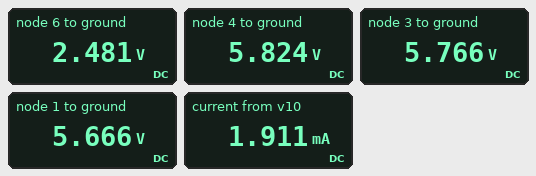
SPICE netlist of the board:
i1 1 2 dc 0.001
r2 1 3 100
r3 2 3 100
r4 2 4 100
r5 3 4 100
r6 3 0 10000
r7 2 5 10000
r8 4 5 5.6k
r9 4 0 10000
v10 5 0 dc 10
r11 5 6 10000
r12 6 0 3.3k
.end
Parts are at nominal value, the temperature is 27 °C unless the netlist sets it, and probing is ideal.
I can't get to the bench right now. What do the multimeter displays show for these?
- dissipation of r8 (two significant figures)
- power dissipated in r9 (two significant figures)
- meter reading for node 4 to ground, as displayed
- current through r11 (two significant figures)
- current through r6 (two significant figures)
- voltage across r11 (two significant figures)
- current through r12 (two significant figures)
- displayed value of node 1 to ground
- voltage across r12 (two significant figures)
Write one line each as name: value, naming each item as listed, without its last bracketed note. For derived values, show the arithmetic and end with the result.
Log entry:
dissipation of r8: (10 V - 5.824 V)^2 / 5.6 kΩ = 3.1 mW
power dissipated in r9: (5.824 V)^2 / 10 kΩ = 3.4 mW
meter reading for node 4 to ground, as displayed: 5.824 V
current through r11: (10 V - 2.481 V) / 10 kΩ = 750 µA
current through r6: (5.766 V) / 10 kΩ = 580 µA
voltage across r11: 10 V - 2.481 V = 7.5 V
current through r12: (2.481 V) / 3.3 kΩ = 750 µA
displayed value of node 1 to ground: 5.666 V
voltage across r12: 2.481 V = 2.5 V
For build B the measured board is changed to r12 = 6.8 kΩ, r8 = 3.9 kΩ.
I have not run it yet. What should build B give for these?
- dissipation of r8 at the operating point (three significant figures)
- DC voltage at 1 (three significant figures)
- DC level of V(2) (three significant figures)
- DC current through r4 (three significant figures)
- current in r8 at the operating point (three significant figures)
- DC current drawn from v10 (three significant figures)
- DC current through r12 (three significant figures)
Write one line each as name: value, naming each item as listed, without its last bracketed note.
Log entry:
dissipation of r8 at the operating point: 3.30 mW
DC voltage at 1: 6.25 V
DC level of V(2): 6.45 V
DC current through r4: 359 µA
current in r8 at the operating point: 920 µA
DC current drawn from v10: 1.87 mA
DC current through r12: 595 µA
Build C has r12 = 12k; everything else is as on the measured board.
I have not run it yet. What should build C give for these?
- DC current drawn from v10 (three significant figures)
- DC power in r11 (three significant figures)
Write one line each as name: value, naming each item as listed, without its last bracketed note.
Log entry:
DC current drawn from v10: 1.61 mA
DC power in r11: 2.07 mW
